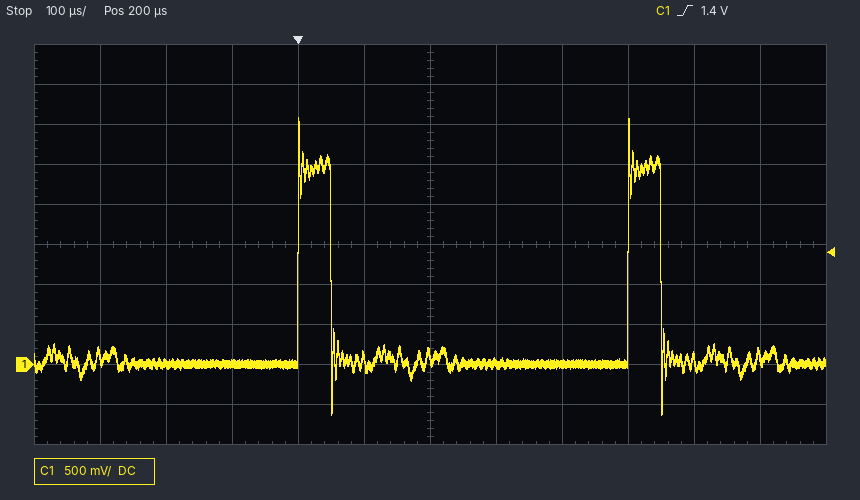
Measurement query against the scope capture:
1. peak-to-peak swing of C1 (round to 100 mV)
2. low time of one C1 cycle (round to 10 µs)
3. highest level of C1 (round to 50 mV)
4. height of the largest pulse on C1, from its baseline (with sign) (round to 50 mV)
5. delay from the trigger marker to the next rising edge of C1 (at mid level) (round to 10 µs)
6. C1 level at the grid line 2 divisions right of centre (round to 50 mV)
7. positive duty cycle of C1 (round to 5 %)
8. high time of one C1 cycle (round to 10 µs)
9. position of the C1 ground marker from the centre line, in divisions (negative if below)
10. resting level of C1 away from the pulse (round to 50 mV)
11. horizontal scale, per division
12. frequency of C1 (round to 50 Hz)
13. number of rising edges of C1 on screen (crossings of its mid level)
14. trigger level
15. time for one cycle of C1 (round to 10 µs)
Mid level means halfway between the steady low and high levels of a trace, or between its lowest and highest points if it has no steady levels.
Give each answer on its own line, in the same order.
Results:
3.70 V
450 µs
3.10 V
+3.10 V
500 µs
0 mV
10 %
50 µs
-3.0 div
0 mV
100 µs
2.00 kHz
2
1.4 V
500 µs
